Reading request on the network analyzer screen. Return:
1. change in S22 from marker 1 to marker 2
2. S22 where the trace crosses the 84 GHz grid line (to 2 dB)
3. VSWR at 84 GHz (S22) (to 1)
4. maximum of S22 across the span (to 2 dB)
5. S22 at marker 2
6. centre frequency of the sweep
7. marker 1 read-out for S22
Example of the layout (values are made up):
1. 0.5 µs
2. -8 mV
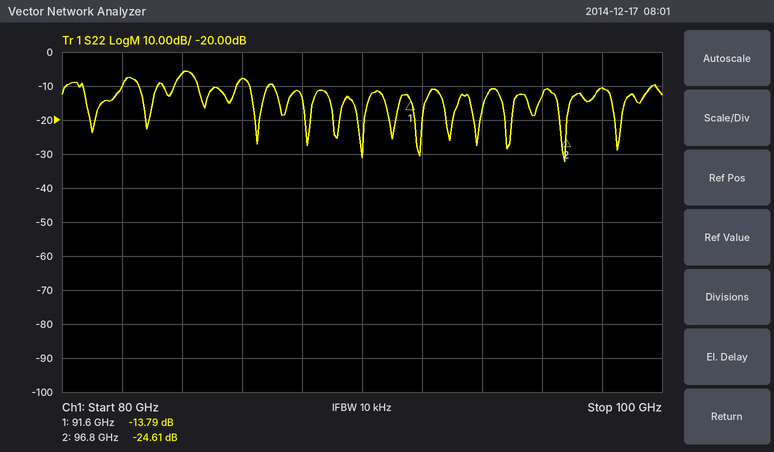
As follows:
1. -10.82 dB
2. -6 dB
3. 3
4. -6 dB
5. -24.61 dB
6. 90 GHz
7. -13.79 dB
